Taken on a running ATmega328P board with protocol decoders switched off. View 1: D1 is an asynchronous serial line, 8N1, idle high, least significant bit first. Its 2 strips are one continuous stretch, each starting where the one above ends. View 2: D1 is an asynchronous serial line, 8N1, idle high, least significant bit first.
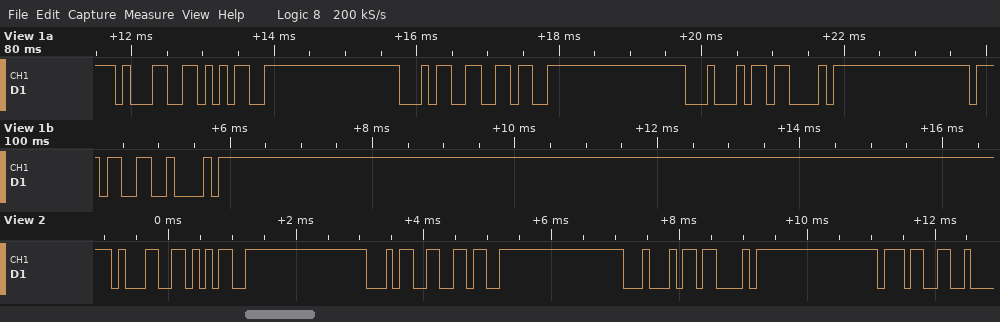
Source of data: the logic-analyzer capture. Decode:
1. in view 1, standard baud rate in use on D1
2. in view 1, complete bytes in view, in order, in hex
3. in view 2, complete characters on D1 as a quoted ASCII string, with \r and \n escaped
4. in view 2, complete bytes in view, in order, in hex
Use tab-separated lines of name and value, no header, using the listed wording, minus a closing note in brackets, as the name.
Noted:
in view 1, standard baud rate in use on D1	9600 baud
in view 1, complete bytes in view, in order, in hex	31 35 34 36 44 43 37 42
in view 2, complete characters on D1 as a quoted ASCII string, with \r and \n escaped	"1546DC7"
in view 2, complete bytes in view, in order, in hex	31 35 34 36 44 43 37
